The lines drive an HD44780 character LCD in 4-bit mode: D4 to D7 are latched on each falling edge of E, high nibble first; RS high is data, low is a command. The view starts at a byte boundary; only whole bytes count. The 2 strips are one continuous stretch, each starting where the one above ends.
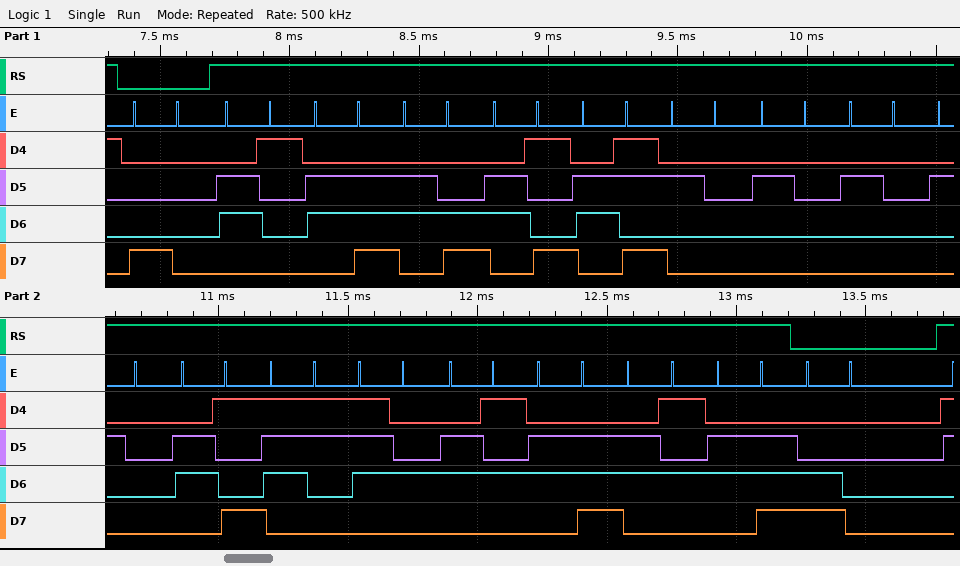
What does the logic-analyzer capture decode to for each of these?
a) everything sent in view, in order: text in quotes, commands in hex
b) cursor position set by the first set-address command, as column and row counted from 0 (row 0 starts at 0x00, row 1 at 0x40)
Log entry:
0x80 "anlik    istenen" 0xC0
column 0, row 0
